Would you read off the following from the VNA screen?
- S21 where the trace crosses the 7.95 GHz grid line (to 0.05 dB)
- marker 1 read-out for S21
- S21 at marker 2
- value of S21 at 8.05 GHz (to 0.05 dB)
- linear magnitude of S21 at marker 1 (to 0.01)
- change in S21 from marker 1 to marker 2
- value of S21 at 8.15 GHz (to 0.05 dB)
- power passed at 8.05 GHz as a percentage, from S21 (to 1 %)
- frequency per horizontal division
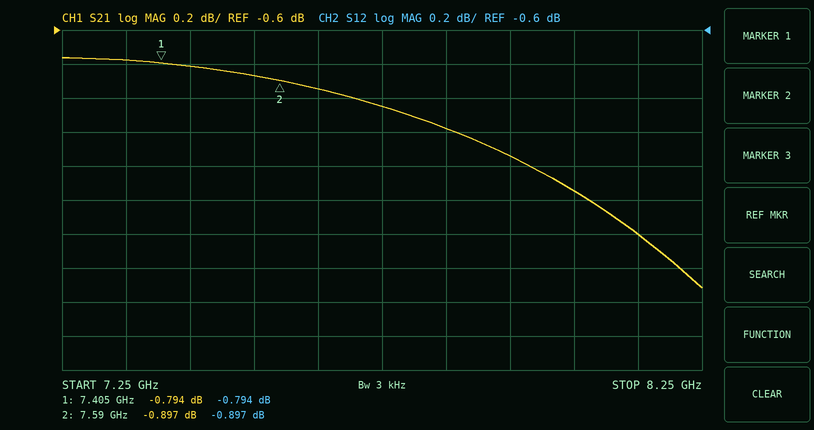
-1.35 dB
-0.794 dB
-0.897 dB
-1.55 dB
0.91
-0.103 dB
-1.80 dB
70 %
100 MHz
